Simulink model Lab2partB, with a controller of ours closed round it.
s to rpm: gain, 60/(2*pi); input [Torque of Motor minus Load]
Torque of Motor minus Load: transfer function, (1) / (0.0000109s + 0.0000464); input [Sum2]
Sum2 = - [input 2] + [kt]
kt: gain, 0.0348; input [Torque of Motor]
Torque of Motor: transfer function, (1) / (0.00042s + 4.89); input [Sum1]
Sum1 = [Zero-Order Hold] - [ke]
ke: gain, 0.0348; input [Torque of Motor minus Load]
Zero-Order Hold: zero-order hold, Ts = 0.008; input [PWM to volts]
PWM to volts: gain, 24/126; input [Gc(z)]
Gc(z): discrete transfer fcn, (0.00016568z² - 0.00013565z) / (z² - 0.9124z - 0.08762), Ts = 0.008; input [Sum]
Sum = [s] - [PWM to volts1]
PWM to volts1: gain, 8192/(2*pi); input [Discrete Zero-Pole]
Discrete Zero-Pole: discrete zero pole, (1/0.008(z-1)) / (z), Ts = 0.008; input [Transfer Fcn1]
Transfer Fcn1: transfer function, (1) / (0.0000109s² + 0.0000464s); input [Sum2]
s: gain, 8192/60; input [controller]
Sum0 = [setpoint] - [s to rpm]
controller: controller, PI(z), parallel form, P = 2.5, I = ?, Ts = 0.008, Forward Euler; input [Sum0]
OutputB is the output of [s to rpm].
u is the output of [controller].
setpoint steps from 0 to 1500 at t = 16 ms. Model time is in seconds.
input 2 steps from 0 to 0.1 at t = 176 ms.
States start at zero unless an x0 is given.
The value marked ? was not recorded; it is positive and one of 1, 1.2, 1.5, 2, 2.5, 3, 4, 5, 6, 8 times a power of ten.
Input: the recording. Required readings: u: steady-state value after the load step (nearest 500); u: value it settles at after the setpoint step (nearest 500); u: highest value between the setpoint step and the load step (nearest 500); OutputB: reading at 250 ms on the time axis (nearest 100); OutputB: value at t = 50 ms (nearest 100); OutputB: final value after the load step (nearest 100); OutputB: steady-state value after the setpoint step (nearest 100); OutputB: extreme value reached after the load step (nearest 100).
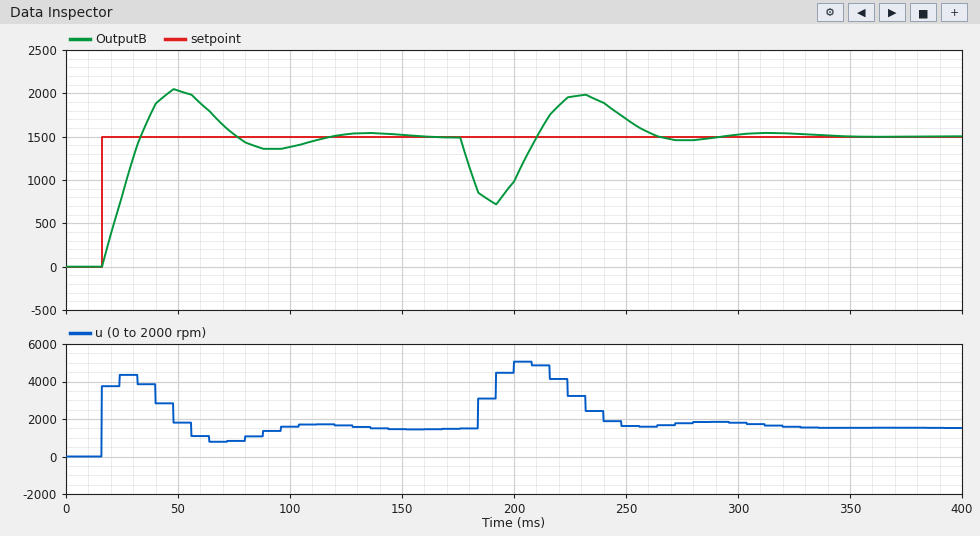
1500
1500
4500
1700
2000
1500
1500
700
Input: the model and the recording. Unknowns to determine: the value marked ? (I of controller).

200
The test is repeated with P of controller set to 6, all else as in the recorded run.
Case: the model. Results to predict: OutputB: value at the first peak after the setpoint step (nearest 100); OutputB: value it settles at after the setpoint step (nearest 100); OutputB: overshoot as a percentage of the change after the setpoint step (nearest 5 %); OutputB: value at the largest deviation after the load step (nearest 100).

1700
1500
15 %
900
